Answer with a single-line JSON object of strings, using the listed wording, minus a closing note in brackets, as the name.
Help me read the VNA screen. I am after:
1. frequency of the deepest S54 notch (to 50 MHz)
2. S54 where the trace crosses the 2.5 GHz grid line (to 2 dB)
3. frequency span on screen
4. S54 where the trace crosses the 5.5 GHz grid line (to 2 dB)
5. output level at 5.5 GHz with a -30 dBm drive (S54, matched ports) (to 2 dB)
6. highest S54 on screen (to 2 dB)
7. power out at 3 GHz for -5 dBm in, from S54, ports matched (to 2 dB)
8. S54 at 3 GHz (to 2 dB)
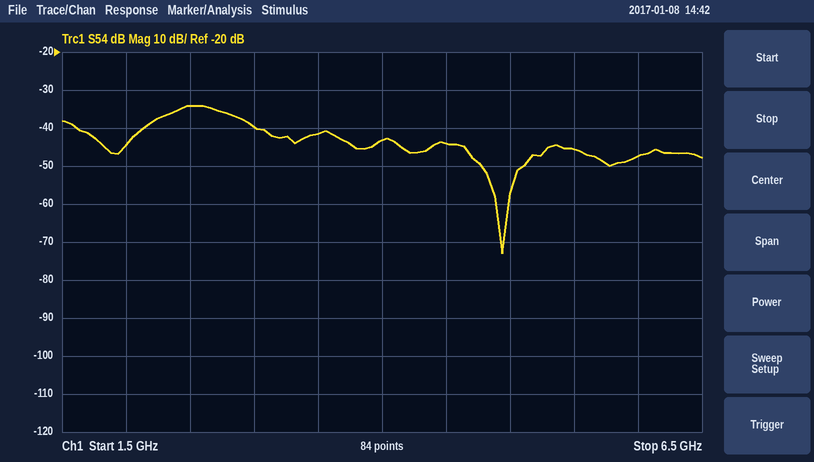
{"frequency of the deepest S54 notch": "4.95 GHz", "S54 where the trace crosses the 2.5 GHz grid line": "-34 dB", "frequency span on screen": "5 GHz", "S54 where the trace crosses the 5.5 GHz grid line": "-46 dB", "output level at 5.5 GHz with a -30 dBm drive (S54, matched ports)": "-76 dBm", "highest S54 on screen": "-34 dB", "power out at 3 GHz for -5 dBm in, from S54, ports matched": "-44 dBm", "S54 at 3 GHz": "-40 dB"}
